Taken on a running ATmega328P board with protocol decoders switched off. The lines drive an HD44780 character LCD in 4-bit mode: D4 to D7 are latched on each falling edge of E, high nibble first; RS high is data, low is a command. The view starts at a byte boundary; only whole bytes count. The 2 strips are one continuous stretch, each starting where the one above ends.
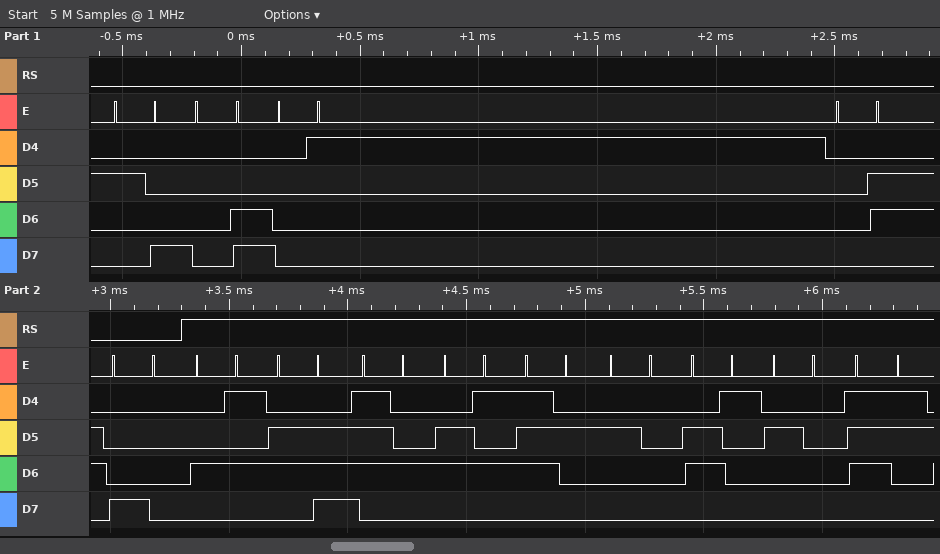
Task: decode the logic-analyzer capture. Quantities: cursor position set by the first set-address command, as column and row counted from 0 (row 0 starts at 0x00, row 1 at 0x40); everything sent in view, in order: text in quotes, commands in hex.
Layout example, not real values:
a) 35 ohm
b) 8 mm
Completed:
a) column 0, row 0
b) 0x28 0x0C 0x01 0x06 0x80 "Enter a s"
